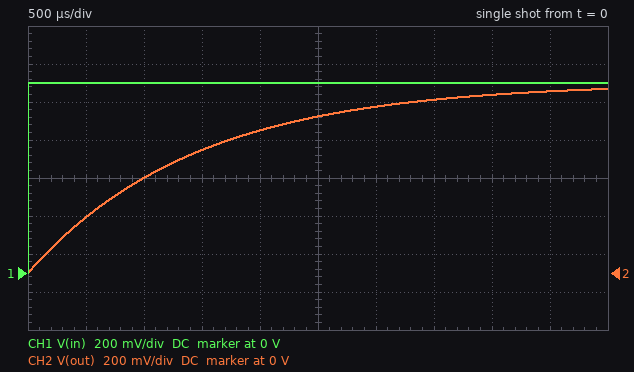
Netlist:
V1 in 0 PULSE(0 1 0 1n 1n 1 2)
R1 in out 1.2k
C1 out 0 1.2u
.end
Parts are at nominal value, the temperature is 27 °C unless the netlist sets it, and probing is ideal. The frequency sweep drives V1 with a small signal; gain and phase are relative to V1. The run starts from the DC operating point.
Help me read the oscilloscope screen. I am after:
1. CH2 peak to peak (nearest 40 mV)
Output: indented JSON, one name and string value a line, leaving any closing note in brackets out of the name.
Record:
{
  "CH2 peak to peak": "960 mV"
}
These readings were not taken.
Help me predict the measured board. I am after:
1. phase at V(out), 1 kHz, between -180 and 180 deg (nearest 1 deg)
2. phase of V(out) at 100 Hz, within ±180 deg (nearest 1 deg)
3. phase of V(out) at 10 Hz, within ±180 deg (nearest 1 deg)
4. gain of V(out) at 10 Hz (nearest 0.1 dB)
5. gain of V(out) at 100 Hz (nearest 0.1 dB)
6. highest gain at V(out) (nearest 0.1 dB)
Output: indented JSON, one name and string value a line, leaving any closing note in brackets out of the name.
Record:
{
  "phase at V(out), 1 kHz, between -180 and 180 deg": "-84 deg",
  "phase of V(out) at 100 Hz, within ±180 deg": "-42 deg",
  "phase of V(out) at 10 Hz, within ±180 deg": "-5 deg",
  "gain of V(out) at 10 Hz": "0 dB",
  "gain of V(out) at 100 Hz": "-2.6 dB",
  "highest gain at V(out)": "0 dB"
}
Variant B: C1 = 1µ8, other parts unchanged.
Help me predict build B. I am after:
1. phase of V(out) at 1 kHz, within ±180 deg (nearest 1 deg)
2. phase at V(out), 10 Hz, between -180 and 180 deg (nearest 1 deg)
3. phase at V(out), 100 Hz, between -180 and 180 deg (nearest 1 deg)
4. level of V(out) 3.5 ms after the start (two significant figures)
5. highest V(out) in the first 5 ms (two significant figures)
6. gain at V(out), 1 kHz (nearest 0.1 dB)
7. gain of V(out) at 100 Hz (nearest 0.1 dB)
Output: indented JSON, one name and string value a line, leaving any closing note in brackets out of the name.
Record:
{
  "phase of V(out) at 1 kHz, within ±180 deg": "-86 deg",
  "phase at V(out), 10 Hz, between -180 and 180 deg": "-8 deg",
  "phase at V(out), 100 Hz, between -180 and 180 deg": "-54 deg",
  "level of V(out) 3.5 ms after the start": "800 mV",
  "highest V(out) in the first 5 ms": "900 mV",
  "gain at V(out), 1 kHz": "-22.7 dB",
  "gain of V(out) at 100 Hz": "-4.5 dB"
}
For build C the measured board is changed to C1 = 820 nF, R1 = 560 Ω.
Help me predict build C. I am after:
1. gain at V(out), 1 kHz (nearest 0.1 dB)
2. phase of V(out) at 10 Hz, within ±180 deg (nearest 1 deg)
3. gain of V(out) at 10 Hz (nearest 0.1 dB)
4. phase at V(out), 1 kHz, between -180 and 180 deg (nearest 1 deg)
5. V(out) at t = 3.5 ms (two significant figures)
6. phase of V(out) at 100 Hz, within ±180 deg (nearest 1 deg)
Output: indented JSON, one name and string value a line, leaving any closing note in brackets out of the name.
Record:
{
  "gain at V(out), 1 kHz": "-9.7 dB",
  "phase of V(out) at 10 Hz, within ±180 deg": "-2 deg",
  "gain of V(out) at 10 Hz": "0 dB",
  "phase at V(out), 1 kHz, between -180 and 180 deg": "-71 deg",
  "V(out) at t = 3.5 ms": "1.0 V",
  "phase of V(out) at 100 Hz, within ±180 deg": "-16 deg"
}
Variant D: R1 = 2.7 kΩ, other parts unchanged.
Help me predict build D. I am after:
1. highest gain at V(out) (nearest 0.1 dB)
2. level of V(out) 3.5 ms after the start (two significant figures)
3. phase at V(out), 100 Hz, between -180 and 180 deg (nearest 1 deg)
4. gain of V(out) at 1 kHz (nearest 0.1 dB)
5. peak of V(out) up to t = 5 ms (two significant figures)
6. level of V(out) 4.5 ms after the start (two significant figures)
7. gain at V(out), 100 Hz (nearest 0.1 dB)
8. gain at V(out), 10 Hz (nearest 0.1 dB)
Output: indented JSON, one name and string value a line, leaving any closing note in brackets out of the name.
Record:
{
  "highest gain at V(out)": "0 dB",
  "level of V(out) 3.5 ms after the start": "660 mV",
  "phase at V(out), 100 Hz, between -180 and 180 deg": "-64 deg",
  "gain of V(out) at 1 kHz": "-26.2 dB",
  "peak of V(out) up to t = 5 ms": "790 mV",
  "level of V(out) 4.5 ms after the start": "750 mV",
  "gain at V(out), 100 Hz": "-7.1 dB",
  "gain at V(out), 10 Hz": "-0.2 dB"
}
